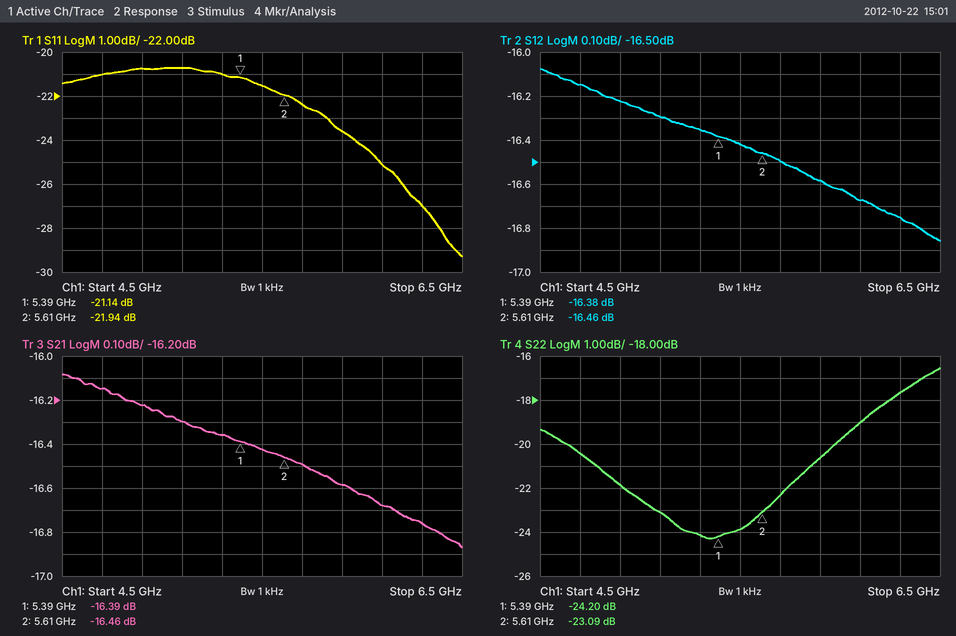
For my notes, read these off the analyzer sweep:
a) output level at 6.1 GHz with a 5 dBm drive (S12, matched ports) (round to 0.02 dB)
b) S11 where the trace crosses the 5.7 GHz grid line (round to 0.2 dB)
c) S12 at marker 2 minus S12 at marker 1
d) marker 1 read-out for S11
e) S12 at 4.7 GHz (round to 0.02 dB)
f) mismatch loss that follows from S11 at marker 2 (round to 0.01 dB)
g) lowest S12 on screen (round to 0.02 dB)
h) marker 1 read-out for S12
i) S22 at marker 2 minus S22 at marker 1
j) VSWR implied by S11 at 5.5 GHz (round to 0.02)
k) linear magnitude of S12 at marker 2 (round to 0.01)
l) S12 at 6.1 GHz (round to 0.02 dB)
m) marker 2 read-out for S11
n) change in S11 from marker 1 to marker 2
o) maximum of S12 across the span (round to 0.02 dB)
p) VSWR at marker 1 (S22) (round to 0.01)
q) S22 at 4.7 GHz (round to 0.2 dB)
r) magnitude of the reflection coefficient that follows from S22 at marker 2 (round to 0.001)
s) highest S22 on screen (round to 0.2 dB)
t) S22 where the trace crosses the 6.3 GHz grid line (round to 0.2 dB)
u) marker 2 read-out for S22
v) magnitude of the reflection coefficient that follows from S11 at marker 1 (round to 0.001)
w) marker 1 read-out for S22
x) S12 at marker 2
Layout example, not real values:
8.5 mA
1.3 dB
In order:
-11.68 dBm
-22.4 dB
-0.08 dB
-21.14 dB
-16.14 dB
0.03 dB
-16.86 dB
-16.38 dB
1.11 dB
1.18
0.15
-16.68 dB
-21.94 dB
-0.80 dB
-16.08 dB
1.13
-20.4 dB
0.070
-16.6 dB
-17.6 dB
-23.09 dB
0.088
-24.20 dB
-16.46 dB
